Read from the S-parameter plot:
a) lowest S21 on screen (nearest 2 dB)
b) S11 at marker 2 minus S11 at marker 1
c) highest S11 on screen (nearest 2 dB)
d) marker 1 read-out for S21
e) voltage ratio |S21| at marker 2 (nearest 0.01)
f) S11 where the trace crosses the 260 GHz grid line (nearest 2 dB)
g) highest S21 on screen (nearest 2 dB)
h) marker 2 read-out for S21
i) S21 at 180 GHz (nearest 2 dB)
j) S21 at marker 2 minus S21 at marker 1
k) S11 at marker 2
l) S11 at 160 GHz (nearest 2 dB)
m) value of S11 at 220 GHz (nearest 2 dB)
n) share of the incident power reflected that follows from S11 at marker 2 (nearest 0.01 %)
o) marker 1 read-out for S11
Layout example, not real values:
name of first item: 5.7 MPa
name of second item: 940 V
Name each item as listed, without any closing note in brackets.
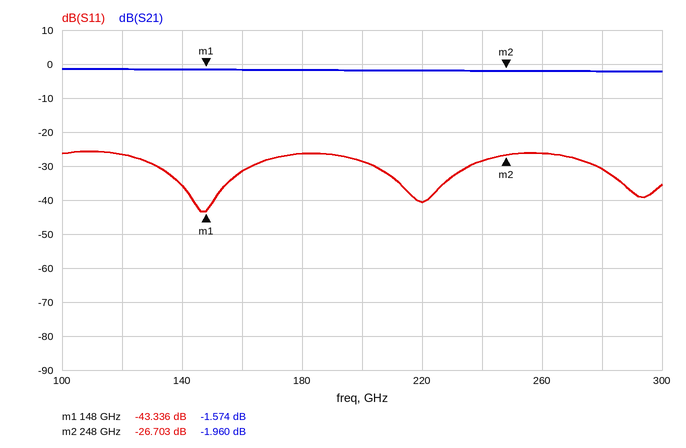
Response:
lowest S21 on screen: -2 dB
S11 at marker 2 minus S11 at marker 1: 16.633 dB
highest S11 on screen: -26 dB
marker 1 read-out for S21: -1.574 dB
voltage ratio |S21| at marker 2: 0.80
S11 where the trace crosses the 260 GHz grid line: -26 dB
highest S21 on screen: -2 dB
marker 2 read-out for S21: -1.960 dB
S21 at 180 GHz: -2 dB
S21 at marker 2 minus S21 at marker 1: -0.386 dB
S11 at marker 2: -26.703 dB
S11 at 160 GHz: -32 dB
value of S11 at 220 GHz: -40 dB
share of the incident power reflected that follows from S11 at marker 2: 0.21 %
marker 1 read-out for S11: -43.336 dB
